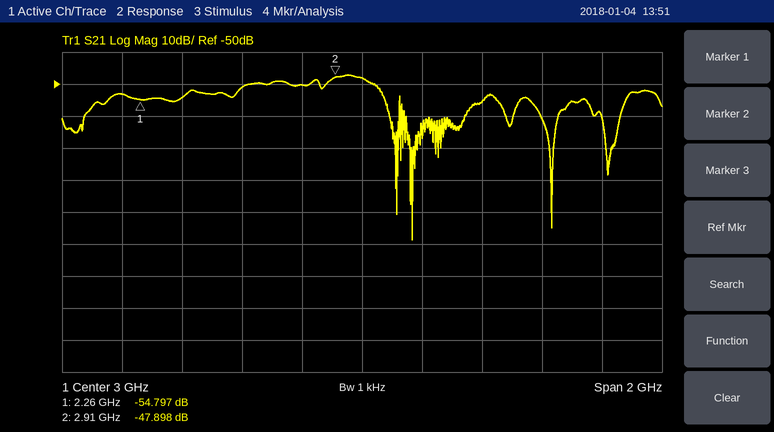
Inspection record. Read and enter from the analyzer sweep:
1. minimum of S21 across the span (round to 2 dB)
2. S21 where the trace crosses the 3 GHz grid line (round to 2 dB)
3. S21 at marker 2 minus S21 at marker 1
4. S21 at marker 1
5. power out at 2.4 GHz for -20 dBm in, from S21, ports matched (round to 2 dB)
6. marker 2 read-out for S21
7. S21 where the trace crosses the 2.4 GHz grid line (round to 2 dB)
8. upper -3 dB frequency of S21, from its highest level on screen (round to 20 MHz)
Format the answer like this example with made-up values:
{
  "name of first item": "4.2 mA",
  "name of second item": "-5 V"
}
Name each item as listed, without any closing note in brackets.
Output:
{
  "minimum of S21 across the span": "-98 dB",
  "S21 where the trace crosses the 3 GHz grid line": "-48 dB",
  "S21 at marker 2 minus S21 at marker 1": "6.899 dB",
  "S21 at marker 1": "-54.797 dB",
  "power out at 2.4 GHz for -20 dBm in, from S21, ports matched": "-74 dBm",
  "marker 2 read-out for S21": "-47.898 dB",
  "S21 where the trace crosses the 2.4 GHz grid line": "-54 dB",
  "upper -3 dB frequency of S21, from its highest level on screen": "3.04 GHz"
}
